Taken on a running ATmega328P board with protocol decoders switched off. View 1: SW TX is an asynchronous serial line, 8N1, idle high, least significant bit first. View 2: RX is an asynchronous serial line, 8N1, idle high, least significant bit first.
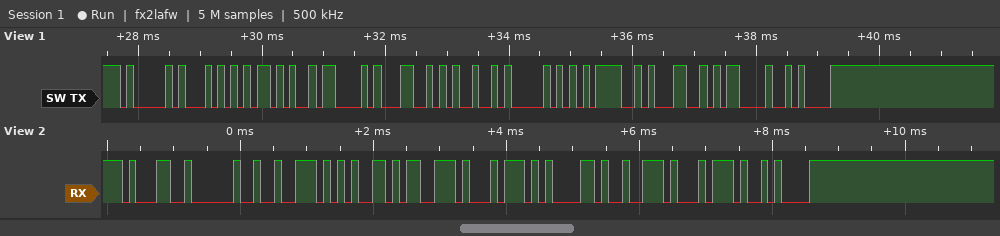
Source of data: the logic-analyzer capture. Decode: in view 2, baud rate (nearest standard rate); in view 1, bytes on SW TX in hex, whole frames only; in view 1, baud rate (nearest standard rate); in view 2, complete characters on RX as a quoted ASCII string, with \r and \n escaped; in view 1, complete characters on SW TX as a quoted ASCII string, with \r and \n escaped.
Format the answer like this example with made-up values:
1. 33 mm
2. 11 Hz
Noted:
1. 9600 baud
2. 0x41 0x54 0x2B 0x43 0x4C 0x49 0x50 0x3D 0x31 0x0D 0x0A
3. 9600 baud
4. "1 restart\n"
5. "AT+CLIP=1\r\n"
